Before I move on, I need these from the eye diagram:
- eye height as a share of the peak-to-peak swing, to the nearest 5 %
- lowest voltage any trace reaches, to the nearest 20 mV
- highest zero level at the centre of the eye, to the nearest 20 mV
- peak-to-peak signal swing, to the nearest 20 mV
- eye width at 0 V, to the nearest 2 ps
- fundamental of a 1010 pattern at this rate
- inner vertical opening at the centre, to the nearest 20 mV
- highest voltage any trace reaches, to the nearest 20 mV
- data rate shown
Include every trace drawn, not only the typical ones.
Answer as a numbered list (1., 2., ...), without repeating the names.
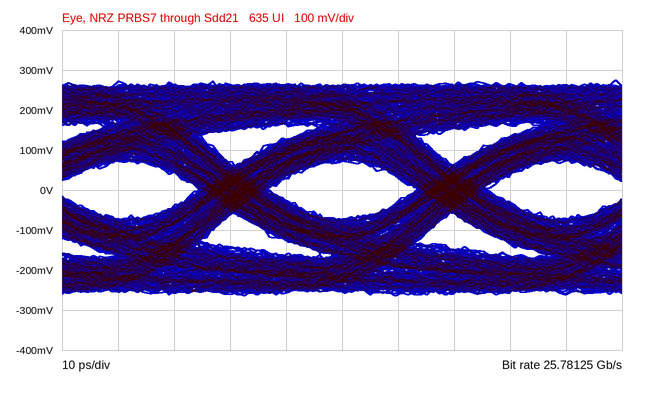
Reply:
1. 25 %
2. -260 mV
3. -80 mV
4. 540 mV
5. 26 ps
6. 12.89062 GHz
7. 140 mV
8. 280 mV
9. 25.78125 Gb/s
